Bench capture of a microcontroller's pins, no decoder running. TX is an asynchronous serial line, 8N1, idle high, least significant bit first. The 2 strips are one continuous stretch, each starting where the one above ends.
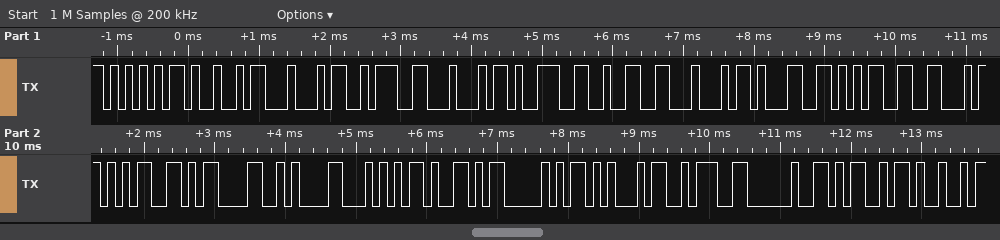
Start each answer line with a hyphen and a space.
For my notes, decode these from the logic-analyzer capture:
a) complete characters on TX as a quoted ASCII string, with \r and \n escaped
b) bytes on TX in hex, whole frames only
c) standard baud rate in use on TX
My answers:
- "UID:D92D15F5\r\nTYPE: MI"
- 55 49 44 3A 44 39 32 44 31 35 46 35 0D 0A 54 59 50 45 3A 20 4D 49
- 9600 baud
